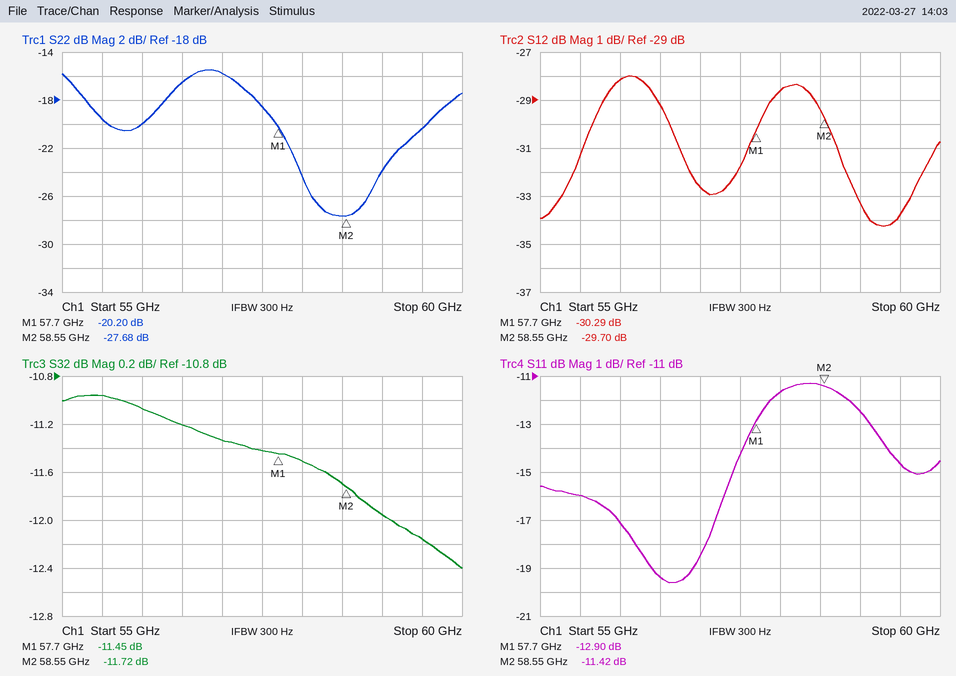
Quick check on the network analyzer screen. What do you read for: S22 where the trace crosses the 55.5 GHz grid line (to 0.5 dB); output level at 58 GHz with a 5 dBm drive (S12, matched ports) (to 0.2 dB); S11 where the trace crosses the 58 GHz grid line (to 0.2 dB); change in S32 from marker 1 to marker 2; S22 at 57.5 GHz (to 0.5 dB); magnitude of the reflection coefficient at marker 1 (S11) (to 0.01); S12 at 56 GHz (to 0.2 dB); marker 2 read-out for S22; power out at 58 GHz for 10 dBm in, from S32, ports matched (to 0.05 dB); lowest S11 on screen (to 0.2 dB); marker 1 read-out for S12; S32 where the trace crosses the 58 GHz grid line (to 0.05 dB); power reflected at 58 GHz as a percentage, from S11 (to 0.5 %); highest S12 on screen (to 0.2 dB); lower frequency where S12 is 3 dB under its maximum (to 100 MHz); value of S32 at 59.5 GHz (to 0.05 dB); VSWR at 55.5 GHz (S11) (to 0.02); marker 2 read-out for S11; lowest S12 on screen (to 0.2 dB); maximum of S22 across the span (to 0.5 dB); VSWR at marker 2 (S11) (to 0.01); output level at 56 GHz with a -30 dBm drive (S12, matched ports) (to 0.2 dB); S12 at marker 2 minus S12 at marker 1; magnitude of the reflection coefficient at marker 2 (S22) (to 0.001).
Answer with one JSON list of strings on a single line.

["-19.5 dB", "-23.6 dBm", "-11.6 dB", "-0.27 dB", "-18.5 dB", "0.23", "-28.2 dB", "-27.68 dB", "-1.50 dBm", "-19.6 dB", "-30.29 dB", "-11.50 dB", "7.0 %", "-28.0 dB", "55.5 GHz", "-12.15 dB", "1.38", "-11.42 dB", "-34.2 dB", "-15.5 dB", "1.73", "-58.2 dBm", "0.59 dB", "0.041"]
